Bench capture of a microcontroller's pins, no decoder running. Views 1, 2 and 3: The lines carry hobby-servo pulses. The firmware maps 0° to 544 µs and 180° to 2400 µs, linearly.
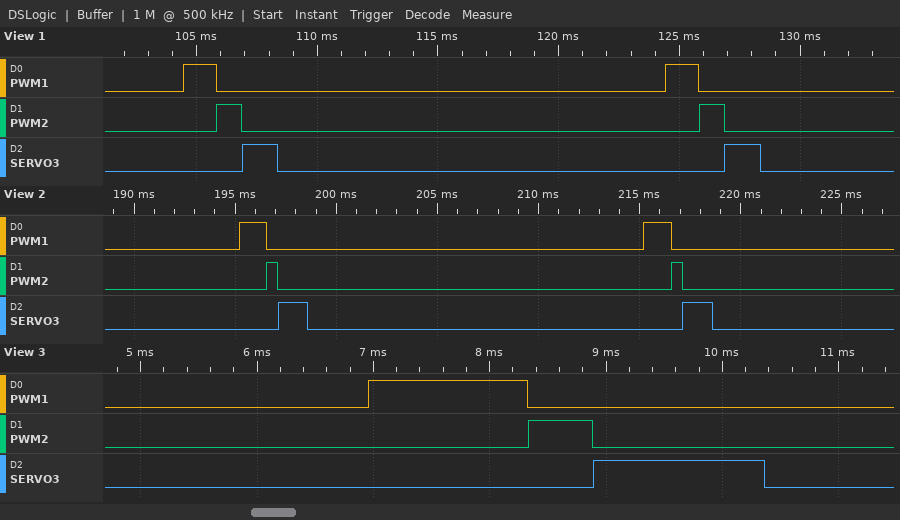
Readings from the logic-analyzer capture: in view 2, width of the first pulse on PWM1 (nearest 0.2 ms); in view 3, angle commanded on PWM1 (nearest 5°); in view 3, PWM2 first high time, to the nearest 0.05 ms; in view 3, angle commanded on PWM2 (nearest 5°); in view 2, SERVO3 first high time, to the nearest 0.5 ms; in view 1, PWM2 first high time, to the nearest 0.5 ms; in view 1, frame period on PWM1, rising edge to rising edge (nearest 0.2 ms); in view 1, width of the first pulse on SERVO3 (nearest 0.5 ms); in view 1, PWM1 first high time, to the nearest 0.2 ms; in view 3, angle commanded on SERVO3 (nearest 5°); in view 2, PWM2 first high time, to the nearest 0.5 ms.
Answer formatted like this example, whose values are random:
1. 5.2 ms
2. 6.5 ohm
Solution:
1. 1.4 ms
2. 80°
3. 0.55 ms
4. 0°
5. 1.5 ms
6. 1.0 ms
7. 20.0 ms
8. 1.5 ms
9. 1.4 ms
10. 90°
11. 0.5 ms
